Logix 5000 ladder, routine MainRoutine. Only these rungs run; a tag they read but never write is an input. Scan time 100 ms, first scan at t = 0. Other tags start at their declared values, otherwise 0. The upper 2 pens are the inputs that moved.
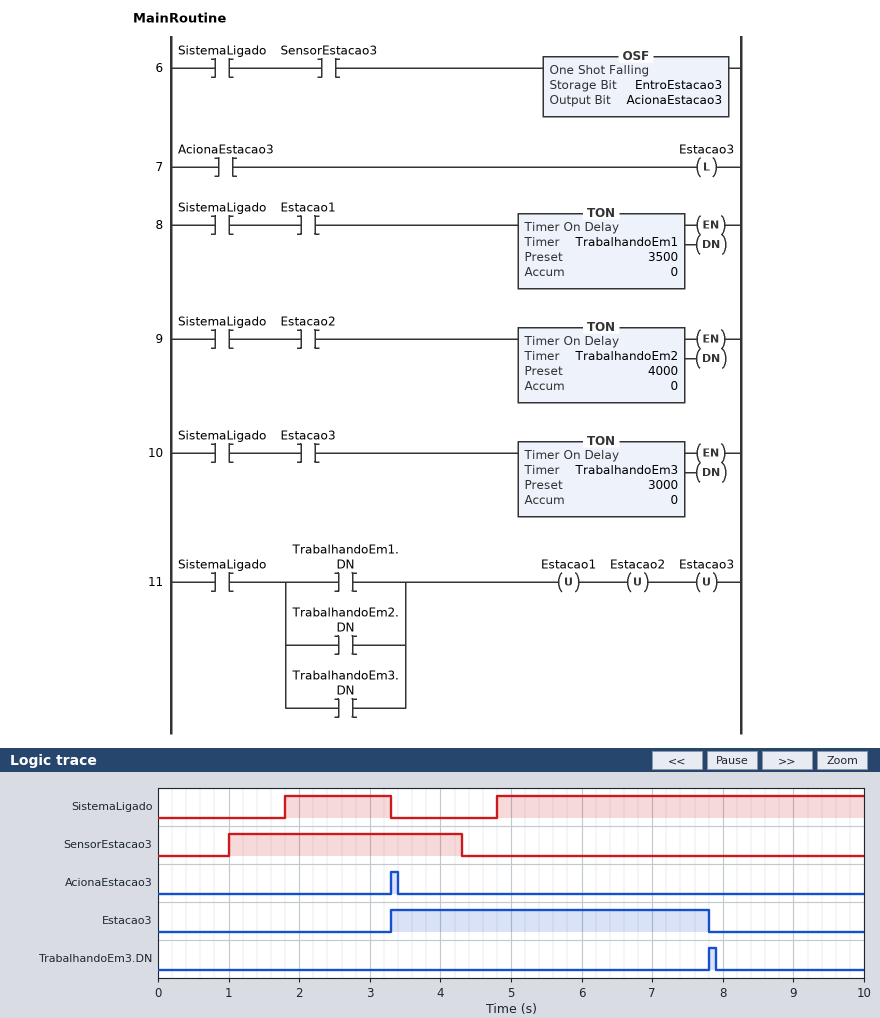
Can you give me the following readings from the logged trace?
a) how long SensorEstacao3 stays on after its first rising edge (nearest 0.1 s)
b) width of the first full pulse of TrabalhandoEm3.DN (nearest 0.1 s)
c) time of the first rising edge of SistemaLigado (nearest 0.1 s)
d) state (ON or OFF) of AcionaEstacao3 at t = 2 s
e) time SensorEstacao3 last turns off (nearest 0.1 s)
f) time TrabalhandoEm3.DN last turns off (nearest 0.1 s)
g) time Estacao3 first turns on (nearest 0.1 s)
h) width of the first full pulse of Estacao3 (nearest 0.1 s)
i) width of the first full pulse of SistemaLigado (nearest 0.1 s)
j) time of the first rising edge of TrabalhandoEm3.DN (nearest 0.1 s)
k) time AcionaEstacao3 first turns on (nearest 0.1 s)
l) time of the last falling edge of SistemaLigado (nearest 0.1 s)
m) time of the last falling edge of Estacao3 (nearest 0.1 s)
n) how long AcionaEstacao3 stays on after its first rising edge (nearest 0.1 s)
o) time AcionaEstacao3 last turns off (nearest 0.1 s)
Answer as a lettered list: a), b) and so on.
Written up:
a) 3.3 s
b) 0.1 s
c) 1.8 s
d) OFF
e) 4.3 s
f) 7.9 s
g) 3.3 s
h) 4.5 s
i) 1.5 s
j) 7.8 s
k) 3.3 s
l) 3.3 s
m) 7.8 s
n) 0.1 s
o) 3.4 s
